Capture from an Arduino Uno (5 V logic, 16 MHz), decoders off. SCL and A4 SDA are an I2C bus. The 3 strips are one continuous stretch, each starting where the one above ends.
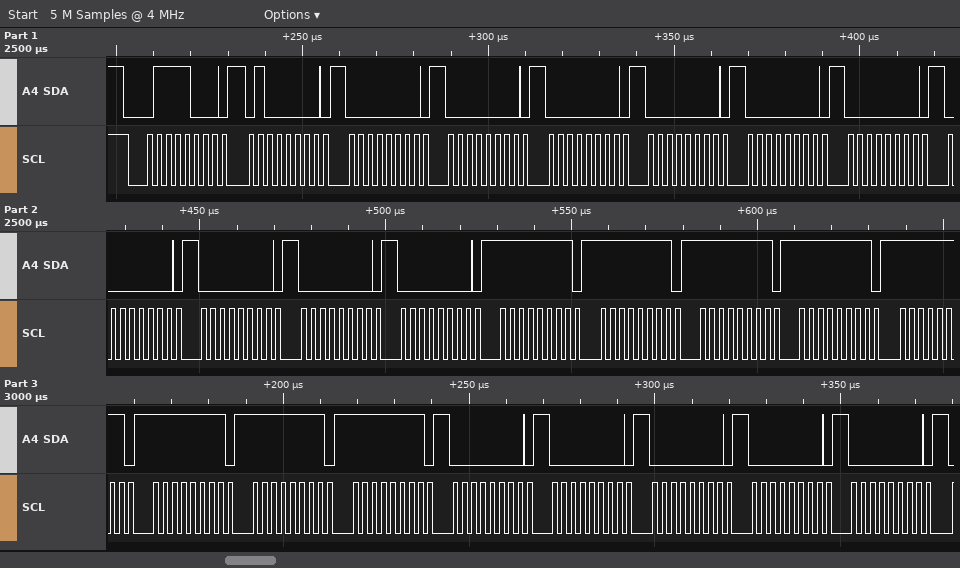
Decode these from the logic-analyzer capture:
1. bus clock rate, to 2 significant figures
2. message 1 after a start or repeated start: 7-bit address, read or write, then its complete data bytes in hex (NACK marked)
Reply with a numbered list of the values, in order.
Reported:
1. 400 kHz
2. 0x3C write: 40 00 00 00 00 00 00 00 00 00 00 FF FF FF FF FF FF FF FF 00 00 00 00 00
